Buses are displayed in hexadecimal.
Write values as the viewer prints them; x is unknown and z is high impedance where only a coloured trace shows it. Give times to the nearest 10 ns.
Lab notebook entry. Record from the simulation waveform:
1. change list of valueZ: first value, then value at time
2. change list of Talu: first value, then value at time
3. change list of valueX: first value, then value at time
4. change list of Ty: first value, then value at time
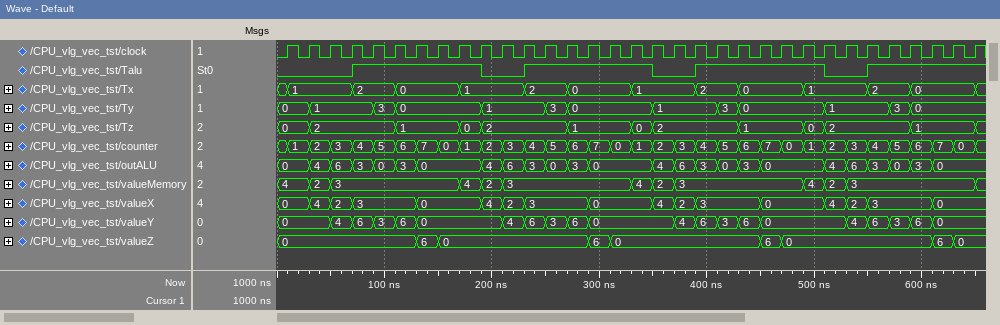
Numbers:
0, 6 at 130 ns, 0 at 150 ns, 6 at 290 ns, 0 at 310 ns, 6 at 450 ns, 0 at 470 ns, 6 at 610 ns, 0 at 630 ns
0, 1 at 70 ns, 0 at 190 ns, 1 at 230 ns, 0 at 350 ns, 1 at 390 ns, 0 at 510 ns, 1 at 550 ns
0, 4 at 30 ns, 2 at 50 ns, 3 at 70 ns, 0 at 130 ns, 4 at 190 ns, 2 at 210 ns, 3 at 230 ns, 0 at 290 ns, 4 at 350 ns, 2 at 370 ns, 3 at 390 ns, 0 at 450 ns, 4 at 510 ns, 2 at 530 ns, 3 at 550 ns, 0 at 610 ns
0, 1 at 30 ns, 3 at 90 ns, 0 at 110 ns, 1 at 190 ns, 3 at 250 ns, 0 at 270 ns, 1 at 350 ns, 3 at 410 ns, 0 at 430 ns, 1 at 510 ns, 3 at 570 ns, 0 at 590 ns
